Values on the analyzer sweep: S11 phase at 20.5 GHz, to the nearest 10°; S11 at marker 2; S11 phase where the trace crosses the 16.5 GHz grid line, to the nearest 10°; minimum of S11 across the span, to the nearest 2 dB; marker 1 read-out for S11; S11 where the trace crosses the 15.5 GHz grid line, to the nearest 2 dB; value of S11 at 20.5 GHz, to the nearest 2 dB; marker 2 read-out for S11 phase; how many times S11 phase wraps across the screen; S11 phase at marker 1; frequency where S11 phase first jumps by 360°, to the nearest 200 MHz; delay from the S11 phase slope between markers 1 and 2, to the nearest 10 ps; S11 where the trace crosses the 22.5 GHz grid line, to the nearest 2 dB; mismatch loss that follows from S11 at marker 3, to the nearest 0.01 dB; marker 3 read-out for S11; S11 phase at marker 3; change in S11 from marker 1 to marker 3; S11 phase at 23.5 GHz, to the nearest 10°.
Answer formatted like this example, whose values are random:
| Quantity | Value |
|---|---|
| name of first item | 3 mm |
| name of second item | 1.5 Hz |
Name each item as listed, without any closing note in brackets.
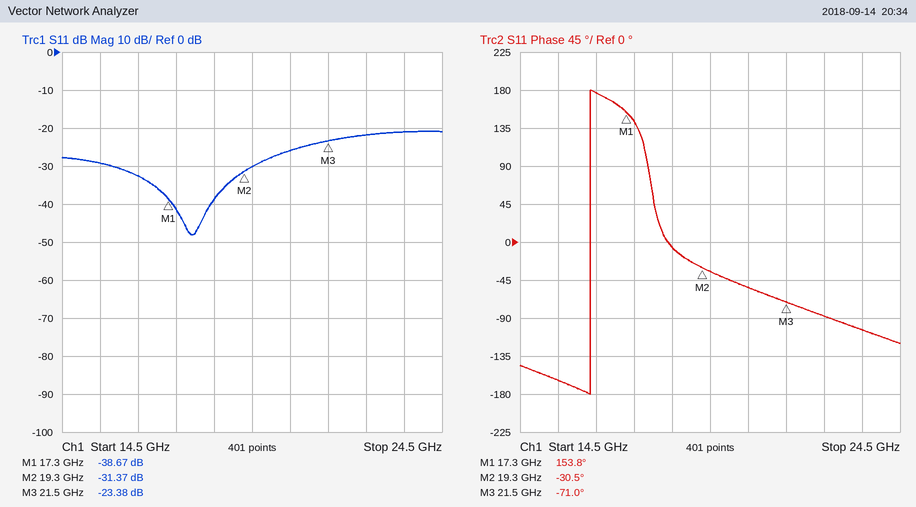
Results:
| Quantity | Value |
|---|---|
| S11 phase at 20.5 GHz, to the nearest 10° | -50° |
| S11 at marker 2 | -31.37 dB |
| S11 phase where the trace crosses the 16.5 GHz grid line, to the nearest 10° | 180° |
| minimum of S11 across the span, to the nearest 2 dB | -48 dB |
| marker 1 read-out for S11 | -38.67 dB |
| S11 where the trace crosses the 15.5 GHz grid line, to the nearest 2 dB | -30 dB |
| value of S11 at 20.5 GHz, to the nearest 2 dB | -26 dB |
| marker 2 read-out for S11 phase | -30.5° |
| how many times S11 phase wraps across the screen | 1 |
| S11 phase at marker 1 | 153.8° |
| frequency where S11 phase first jumps by 360°, to the nearest 200 MHz | 16.4 GHz |
| delay from the S11 phase slope between markers 1 and 2, to the nearest 10 ps | 260 ps |
| S11 where the trace crosses the 22.5 GHz grid line, to the nearest 2 dB | -22 dB |
| mismatch loss that follows from S11 at marker 3, to the nearest 0.01 dB | 0.02 dB |
| marker 3 read-out for S11 | -23.38 dB |
| S11 phase at marker 3 | -71.0° |
| change in S11 from marker 1 to marker 3 | 15.29 dB |
| S11 phase at 23.5 GHz, to the nearest 10° | -100° |
